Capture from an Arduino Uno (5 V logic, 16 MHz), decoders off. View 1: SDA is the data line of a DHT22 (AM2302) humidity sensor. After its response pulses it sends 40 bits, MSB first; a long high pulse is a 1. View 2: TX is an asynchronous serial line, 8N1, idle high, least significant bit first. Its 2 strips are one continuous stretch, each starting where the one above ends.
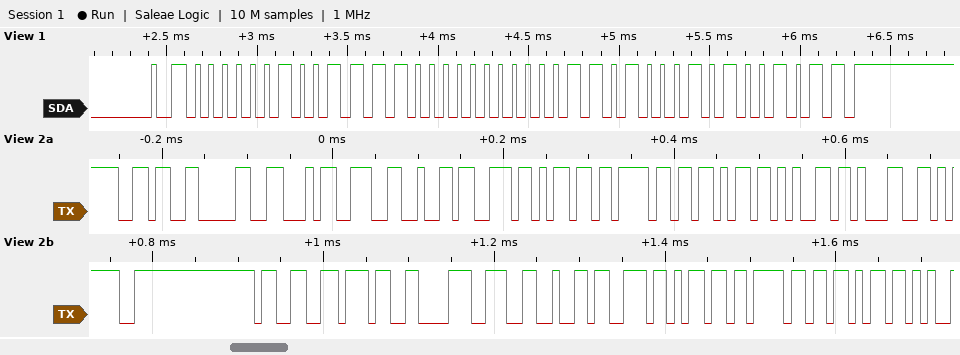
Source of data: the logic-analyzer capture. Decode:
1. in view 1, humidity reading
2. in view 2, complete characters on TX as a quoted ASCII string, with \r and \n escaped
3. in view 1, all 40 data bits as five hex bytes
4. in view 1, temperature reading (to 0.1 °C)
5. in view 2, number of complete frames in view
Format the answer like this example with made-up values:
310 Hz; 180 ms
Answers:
63.2 %; "604&smoke1=378&smok"; 02 78 00 D1 4B; 20.9 °C; 19
